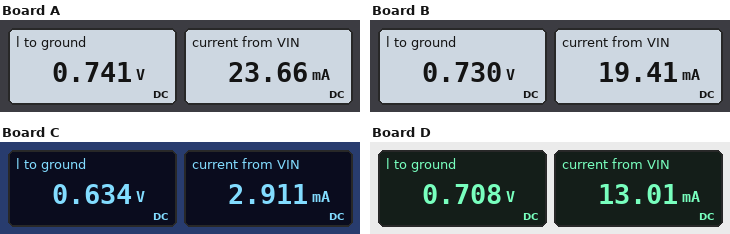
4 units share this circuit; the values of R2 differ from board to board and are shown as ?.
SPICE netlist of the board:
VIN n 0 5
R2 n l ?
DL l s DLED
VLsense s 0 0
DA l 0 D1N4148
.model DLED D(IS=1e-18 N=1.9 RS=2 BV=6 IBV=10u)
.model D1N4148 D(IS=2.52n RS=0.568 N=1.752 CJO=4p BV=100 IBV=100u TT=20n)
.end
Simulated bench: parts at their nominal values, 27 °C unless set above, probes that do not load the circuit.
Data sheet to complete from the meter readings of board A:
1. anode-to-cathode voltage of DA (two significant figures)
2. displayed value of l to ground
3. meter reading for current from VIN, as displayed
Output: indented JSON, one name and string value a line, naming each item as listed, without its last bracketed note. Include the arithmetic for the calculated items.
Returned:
{
  "anode-to-cathode voltage of DA": "741 mV = 740 mV",
  "displayed value of l to ground": "0.741 V",
  "meter reading for current from VIN, as displayed": "23.66 mA"
}
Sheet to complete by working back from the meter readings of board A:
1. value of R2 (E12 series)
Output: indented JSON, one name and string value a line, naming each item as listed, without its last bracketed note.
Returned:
{
  "value of R2": "180 Ω"
}
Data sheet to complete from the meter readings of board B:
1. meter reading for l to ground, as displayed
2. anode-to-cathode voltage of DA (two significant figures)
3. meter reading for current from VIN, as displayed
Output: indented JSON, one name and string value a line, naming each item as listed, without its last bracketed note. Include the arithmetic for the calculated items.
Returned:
{
  "meter reading for l to ground, as displayed": "0.730 V",
  "anode-to-cathode voltage of DA": "730 mV = 730 mV",
  "meter reading for current from VIN, as displayed": "19.41 mA"
}
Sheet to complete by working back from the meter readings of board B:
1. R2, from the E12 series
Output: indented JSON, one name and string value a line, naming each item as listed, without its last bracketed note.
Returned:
{
  "R2, from the E12 series": "220 Ω"
}
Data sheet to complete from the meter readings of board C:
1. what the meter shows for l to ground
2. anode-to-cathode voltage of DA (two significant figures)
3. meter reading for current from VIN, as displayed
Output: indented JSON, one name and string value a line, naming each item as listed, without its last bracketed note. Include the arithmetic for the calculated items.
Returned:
{
  "what the meter shows for l to ground": "0.634 V",
  "anode-to-cathode voltage of DA": "634 mV = 630 mV",
  "meter reading for current from VIN, as displayed": "2.911 mA"
}
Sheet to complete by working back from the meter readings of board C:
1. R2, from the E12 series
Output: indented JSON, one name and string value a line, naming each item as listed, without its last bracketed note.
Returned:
{
  "R2, from the E12 series": "1.5 kΩ"
}
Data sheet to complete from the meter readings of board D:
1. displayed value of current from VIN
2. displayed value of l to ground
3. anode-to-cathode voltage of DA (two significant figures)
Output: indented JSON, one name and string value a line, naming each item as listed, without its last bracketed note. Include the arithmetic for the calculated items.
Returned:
{
  "displayed value of current from VIN": "13.01 mA",
  "displayed value of l to ground": "0.708 V",
  "anode-to-cathode voltage of DA": "708 mV = 710 mV"
}
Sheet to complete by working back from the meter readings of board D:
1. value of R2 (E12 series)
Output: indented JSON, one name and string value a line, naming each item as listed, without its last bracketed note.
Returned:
{
  "value of R2": "330 Ω"
}
